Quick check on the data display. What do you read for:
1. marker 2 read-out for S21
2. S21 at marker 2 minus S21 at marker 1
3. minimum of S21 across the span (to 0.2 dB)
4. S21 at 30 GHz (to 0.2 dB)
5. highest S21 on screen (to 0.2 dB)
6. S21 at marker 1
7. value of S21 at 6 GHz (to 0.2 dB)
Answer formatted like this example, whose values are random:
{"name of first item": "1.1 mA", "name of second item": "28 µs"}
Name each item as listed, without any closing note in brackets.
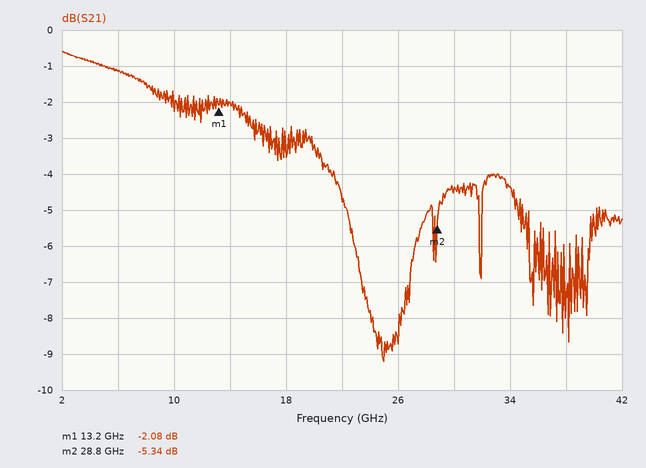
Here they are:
{"marker 2 read-out for S21": "-5.34 dB", "S21 at marker 2 minus S21 at marker 1": "-3.26 dB", "minimum of S21 across the span": "-9.2 dB", "S21 at 30 GHz": "-4.4 dB", "highest S21 on screen": "-0.6 dB", "S21 at marker 1": "-2.08 dB", "value of S21 at 6 GHz": "-1.2 dB"}
